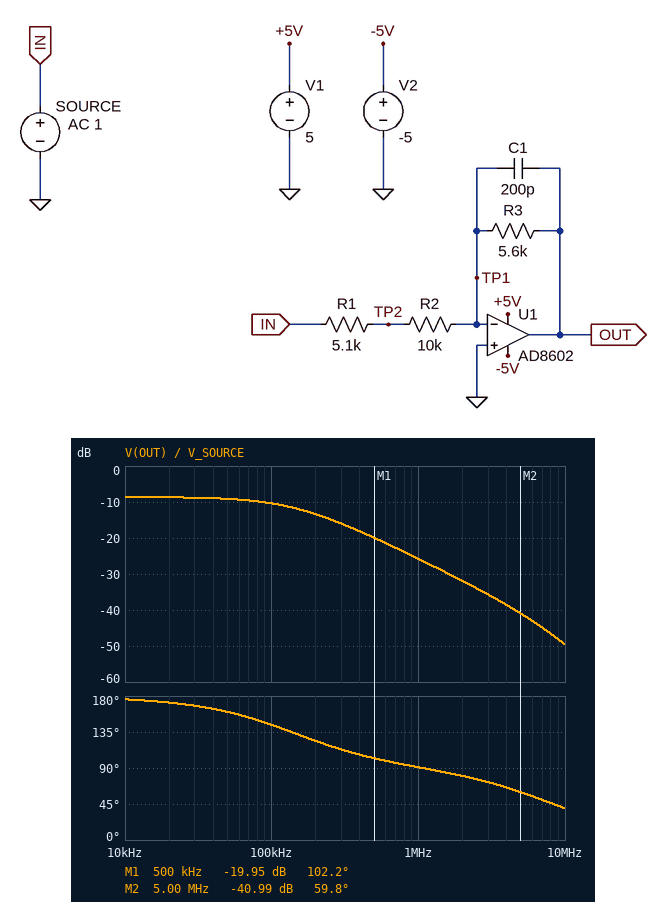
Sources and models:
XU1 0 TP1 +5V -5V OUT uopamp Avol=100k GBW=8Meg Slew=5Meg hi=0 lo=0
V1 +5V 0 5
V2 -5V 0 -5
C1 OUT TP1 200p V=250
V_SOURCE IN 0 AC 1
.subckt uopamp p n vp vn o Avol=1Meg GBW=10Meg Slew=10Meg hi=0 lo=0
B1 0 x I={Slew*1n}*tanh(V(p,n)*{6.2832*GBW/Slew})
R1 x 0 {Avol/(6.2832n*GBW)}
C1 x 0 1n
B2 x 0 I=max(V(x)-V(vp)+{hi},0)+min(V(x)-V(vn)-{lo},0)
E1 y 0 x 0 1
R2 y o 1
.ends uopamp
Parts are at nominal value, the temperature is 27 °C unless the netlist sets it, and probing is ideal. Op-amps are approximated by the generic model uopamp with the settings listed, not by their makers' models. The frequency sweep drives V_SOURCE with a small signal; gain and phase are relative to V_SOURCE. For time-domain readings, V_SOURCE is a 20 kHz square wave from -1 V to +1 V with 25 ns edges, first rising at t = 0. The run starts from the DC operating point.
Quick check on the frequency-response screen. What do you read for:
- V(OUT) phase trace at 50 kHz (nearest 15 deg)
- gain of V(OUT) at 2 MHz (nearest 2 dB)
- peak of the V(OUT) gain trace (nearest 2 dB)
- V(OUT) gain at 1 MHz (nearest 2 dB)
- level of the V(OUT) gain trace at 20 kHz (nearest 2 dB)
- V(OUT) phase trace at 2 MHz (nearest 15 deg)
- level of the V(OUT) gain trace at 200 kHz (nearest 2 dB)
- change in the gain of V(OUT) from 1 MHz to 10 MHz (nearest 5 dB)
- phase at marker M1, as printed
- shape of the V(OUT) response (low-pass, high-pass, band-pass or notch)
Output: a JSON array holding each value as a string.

["165 deg", "-32 dB", "-8 dB", "-26 dB", "-8 dB", "75 deg", "-14 dB", "-25 dB", "102.2 deg", "low-pass"]
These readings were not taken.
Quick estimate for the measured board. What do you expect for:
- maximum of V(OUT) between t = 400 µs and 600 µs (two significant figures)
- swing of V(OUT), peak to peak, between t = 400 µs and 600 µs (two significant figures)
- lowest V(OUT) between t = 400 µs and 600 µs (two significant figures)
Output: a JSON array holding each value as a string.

["370 mV", "740 mV", "-370 mV"]
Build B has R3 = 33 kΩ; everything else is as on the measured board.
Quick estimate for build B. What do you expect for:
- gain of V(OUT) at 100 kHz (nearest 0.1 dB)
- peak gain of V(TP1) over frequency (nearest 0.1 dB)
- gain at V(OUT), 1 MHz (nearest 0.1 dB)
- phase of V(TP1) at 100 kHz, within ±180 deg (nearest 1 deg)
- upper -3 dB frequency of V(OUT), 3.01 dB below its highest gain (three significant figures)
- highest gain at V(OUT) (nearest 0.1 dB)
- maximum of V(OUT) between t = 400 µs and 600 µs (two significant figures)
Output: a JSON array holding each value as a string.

["-5.9 dB", "-43.7 dB", "-25.7 dB", "13 deg", "24.0 kHz", "6.8 dB", "2.1 V"]
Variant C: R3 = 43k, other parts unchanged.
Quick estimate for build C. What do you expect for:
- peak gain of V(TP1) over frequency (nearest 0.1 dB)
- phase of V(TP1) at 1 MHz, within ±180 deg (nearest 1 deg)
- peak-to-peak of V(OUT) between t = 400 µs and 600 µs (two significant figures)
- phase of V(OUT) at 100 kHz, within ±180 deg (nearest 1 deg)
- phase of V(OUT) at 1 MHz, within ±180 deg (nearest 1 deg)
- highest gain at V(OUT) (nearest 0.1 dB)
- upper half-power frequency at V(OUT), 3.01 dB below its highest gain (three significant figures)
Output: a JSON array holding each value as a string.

["-43.7 dB", "-6 deg", "5.1 V", "100 deg", "84 deg", "9.1 dB", "18.4 kHz"]
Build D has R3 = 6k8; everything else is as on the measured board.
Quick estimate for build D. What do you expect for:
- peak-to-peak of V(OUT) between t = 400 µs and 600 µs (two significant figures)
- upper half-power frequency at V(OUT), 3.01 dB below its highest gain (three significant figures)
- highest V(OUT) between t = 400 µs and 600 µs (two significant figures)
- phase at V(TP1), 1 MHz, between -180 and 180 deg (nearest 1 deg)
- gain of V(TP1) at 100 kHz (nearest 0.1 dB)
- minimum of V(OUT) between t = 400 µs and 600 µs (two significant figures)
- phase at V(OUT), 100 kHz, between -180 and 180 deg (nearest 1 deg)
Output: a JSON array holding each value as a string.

["900 mV", "116 kHz", "450 mV", "0 deg", "-47.4 dB", "-450 mV", "139 deg"]
